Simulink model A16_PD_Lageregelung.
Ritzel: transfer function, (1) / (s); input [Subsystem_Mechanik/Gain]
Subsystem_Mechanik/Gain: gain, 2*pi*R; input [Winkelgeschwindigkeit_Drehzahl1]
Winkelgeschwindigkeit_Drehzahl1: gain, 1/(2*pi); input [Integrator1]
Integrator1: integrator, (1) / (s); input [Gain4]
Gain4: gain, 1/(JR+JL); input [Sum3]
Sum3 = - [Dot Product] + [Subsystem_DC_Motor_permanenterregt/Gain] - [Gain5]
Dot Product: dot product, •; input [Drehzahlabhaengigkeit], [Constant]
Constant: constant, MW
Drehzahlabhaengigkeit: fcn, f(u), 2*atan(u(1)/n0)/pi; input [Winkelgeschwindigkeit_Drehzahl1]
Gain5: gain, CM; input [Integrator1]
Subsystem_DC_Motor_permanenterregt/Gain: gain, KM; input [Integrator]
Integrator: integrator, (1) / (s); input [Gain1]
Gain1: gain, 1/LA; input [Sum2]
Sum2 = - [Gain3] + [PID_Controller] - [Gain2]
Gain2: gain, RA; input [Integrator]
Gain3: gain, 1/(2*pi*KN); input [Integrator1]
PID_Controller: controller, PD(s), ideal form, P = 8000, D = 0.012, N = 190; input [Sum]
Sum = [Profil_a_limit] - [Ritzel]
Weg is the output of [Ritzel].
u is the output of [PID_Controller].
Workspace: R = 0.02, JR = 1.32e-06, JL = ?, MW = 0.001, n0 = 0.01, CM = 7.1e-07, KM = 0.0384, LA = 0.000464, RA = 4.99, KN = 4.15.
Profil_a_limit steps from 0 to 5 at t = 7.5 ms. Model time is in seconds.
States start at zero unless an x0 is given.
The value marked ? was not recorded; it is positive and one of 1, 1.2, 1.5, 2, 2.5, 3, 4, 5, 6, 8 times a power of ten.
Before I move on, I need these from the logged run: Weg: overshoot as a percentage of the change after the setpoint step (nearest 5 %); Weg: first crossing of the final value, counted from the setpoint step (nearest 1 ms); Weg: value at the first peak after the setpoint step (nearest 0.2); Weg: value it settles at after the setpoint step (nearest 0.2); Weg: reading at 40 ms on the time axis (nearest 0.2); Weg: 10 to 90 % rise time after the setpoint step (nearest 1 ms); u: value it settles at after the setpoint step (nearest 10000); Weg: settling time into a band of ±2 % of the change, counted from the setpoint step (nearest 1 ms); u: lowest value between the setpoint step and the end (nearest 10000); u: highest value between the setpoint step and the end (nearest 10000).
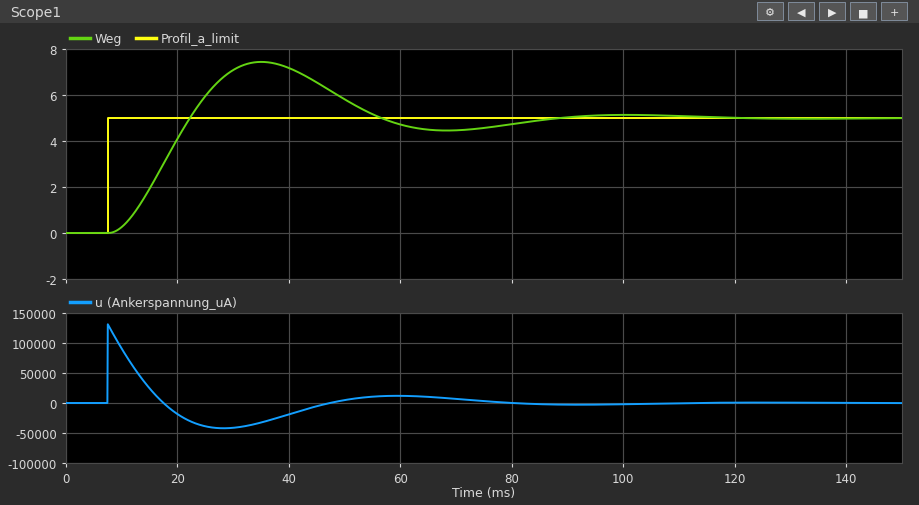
50 %
15 ms
7.4
5.0
7.2
10 ms
0
101 ms
-40000
130000
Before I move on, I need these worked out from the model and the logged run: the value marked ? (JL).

0.0002
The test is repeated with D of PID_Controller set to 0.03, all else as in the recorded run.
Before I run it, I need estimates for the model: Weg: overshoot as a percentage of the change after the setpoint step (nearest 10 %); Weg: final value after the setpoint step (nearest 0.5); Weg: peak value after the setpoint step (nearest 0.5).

40 %
5.0
7.0
